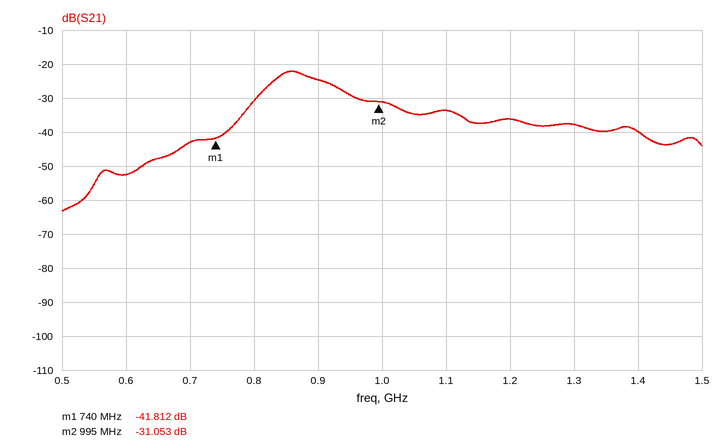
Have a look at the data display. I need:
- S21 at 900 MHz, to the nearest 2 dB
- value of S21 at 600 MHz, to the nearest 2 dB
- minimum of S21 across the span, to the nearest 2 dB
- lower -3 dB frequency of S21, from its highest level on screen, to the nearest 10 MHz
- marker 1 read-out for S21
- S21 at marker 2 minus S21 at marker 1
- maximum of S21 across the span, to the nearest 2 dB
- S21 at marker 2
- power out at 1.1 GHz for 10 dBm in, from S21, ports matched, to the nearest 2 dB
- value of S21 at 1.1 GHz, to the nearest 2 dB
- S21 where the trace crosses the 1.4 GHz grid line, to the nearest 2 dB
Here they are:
-24 dB
-52 dB
-64 dB
830 MHz
-41.812 dB
10.759 dB
-22 dB
-31.053 dB
-24 dBm
-34 dB
-40 dB
